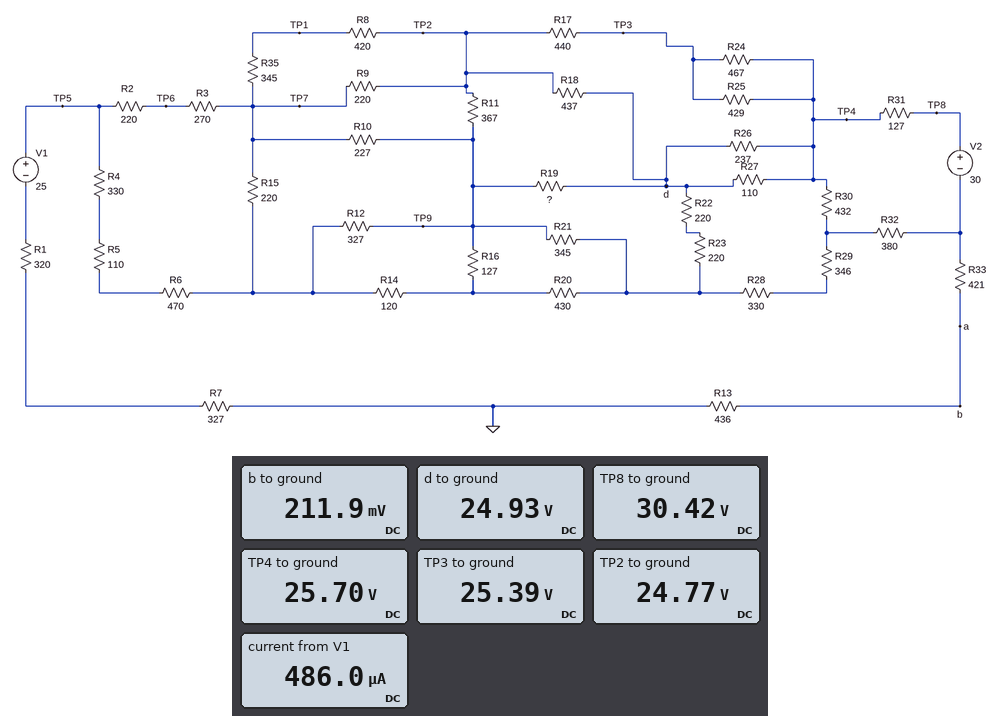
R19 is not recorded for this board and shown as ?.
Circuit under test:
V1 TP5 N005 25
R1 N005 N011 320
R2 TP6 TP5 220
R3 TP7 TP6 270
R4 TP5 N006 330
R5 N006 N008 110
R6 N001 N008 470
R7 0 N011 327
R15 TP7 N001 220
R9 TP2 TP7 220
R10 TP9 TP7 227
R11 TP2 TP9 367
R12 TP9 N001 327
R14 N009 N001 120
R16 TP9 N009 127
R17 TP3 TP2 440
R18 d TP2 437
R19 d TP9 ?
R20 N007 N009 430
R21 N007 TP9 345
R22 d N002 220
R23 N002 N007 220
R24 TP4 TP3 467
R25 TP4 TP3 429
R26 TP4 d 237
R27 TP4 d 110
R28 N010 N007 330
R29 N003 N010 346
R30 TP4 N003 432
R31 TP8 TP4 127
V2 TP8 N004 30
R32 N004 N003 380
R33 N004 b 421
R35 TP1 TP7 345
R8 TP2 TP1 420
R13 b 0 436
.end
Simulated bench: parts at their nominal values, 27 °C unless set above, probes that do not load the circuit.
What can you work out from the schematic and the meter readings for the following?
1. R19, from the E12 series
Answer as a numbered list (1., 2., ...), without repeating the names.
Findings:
1. 82 Ω
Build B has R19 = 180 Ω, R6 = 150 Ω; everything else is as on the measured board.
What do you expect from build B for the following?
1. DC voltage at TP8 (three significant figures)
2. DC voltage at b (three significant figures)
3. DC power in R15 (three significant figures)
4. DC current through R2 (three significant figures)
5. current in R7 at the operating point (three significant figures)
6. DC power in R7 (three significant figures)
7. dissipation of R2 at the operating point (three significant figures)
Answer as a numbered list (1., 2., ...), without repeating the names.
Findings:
1. 30.5 V
2. 267 mV
3. 154 µW
4. 164 µA
5. 613 µA
6. 123 µW
7. 5.95 µW
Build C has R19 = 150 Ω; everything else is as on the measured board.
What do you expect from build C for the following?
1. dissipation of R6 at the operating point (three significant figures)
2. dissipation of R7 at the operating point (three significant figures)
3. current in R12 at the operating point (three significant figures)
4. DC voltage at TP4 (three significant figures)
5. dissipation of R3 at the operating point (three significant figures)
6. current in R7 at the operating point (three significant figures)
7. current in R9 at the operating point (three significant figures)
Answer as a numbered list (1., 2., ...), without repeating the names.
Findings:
1. 52.0 µW
2. 104 µW
3. 138 µA
4. 25.8 V
5. 14.3 µW
6. 563 µA
7. 985 µA
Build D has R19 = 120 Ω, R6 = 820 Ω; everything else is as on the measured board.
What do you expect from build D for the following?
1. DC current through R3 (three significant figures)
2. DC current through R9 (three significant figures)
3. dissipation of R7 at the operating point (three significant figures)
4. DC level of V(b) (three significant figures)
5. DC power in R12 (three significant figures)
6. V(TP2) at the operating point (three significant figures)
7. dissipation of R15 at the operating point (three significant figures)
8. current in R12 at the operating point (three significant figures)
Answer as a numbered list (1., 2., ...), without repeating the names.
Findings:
1. 264 µA
2. 908 µA
3. 87.6 µW
4. 226 mV
5. 11.0 µW
6. 24.7 V
7. 164 µW
8. 184 µA
